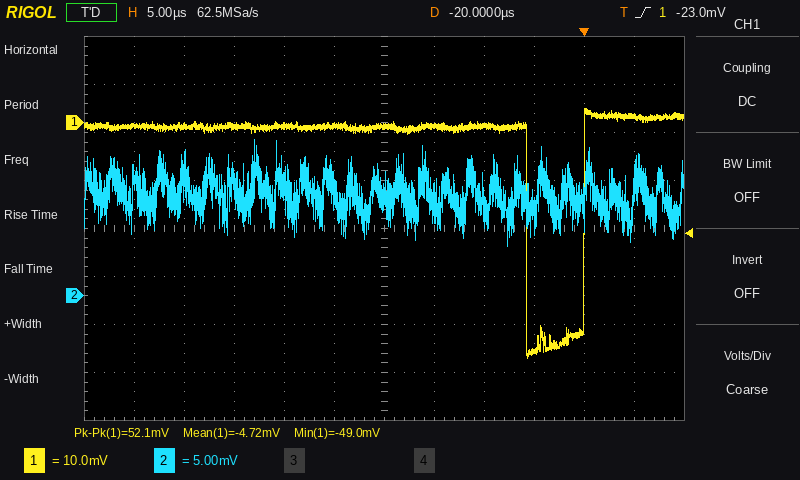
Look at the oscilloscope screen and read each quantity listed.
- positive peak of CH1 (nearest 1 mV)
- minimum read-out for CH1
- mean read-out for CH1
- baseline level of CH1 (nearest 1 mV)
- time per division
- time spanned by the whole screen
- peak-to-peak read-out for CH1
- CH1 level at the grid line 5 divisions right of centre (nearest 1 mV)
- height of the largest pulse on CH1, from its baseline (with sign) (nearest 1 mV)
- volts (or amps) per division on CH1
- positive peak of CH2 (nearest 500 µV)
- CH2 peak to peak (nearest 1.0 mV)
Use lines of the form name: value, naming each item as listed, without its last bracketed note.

positive peak of CH1: 3 mV
minimum read-out for CH1: -49.0 mV
mean read-out for CH1: -4.72 mV
baseline level of CH1: -1 mV
time per division: 5 µs
time spanned by the whole screen: 60 µs
peak-to-peak read-out for CH1: 52.1 mV
CH1 level at the grid line 5 divisions right of centre: 1 mV
height of the largest pulse on CH1, from its baseline (with sign): -48 mV
volts (or amps) per division on CH1: 10 mV
positive peak of CH2: 16.5 mV
CH2 peak to peak: 11.0 mV
